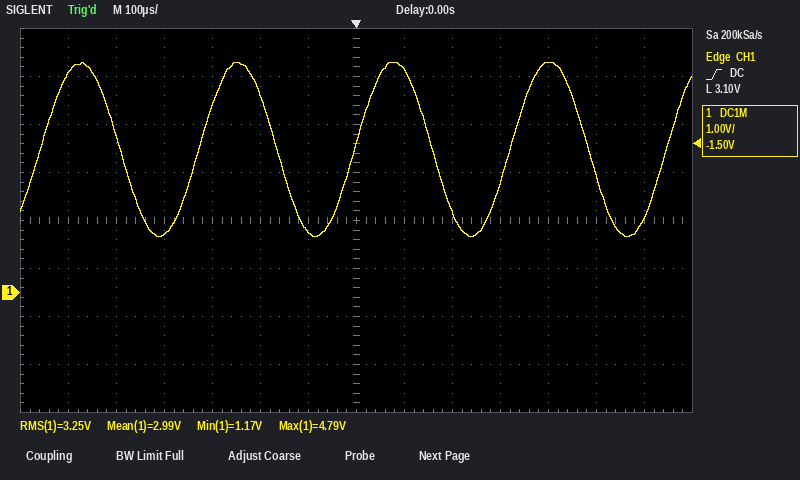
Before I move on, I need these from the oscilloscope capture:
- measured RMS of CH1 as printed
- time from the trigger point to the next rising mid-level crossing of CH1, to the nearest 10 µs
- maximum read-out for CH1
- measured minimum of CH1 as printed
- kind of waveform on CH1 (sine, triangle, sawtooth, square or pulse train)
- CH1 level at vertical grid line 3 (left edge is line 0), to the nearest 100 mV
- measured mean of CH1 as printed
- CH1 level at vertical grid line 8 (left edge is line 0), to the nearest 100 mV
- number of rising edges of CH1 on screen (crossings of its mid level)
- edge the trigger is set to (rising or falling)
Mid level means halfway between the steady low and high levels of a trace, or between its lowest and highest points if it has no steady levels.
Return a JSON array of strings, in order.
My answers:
["3.25 V", "320 µs", "4.79 V", "1.17 V", "sine", "1.2 V", "2.99 V", "4.6 V", "5", "rising"]
